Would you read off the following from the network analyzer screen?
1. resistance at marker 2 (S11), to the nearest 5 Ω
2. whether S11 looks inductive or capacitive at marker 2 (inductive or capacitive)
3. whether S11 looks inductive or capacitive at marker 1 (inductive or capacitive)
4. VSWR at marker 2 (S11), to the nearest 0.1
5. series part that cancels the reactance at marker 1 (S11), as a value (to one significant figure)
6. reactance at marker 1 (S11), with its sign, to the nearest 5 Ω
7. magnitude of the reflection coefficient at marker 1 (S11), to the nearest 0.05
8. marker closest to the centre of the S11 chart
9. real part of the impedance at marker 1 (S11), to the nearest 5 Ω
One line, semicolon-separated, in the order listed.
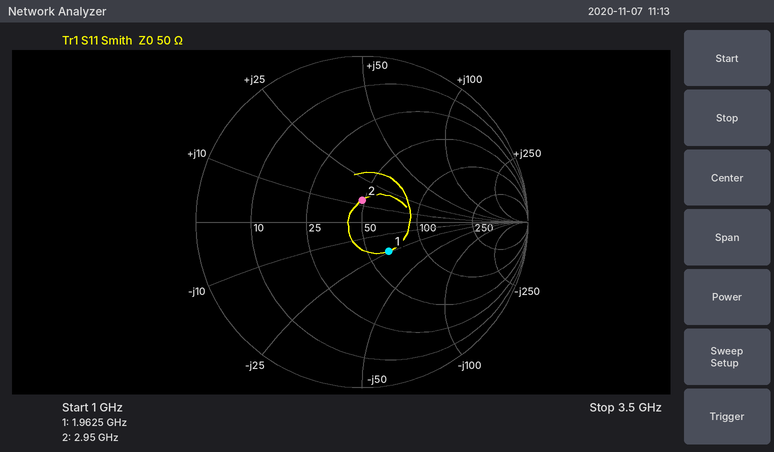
50 Ω; inductive; capacitive; 1.3; 2 nH; -25 Ω; 0.25; marker 2; 65 Ω
